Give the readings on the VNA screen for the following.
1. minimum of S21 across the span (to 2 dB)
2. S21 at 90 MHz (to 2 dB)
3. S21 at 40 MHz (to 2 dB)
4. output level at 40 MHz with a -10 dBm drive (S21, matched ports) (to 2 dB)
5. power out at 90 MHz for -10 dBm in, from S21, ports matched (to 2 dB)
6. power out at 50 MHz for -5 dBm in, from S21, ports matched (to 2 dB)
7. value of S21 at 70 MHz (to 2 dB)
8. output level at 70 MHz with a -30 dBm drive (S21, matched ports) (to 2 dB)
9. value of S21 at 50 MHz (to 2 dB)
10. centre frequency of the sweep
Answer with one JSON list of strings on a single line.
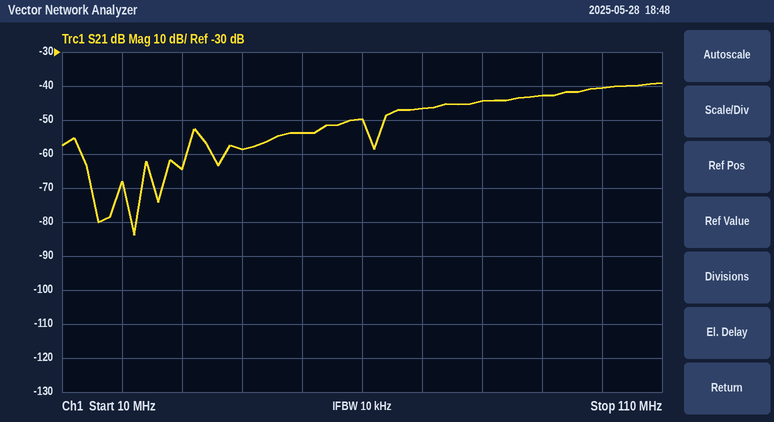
["-84 dB", "-42 dB", "-58 dB", "-68 dBm", "-52 dBm", "-58 dBm", "-46 dB", "-76 dBm", "-54 dB", "60 MHz"]
